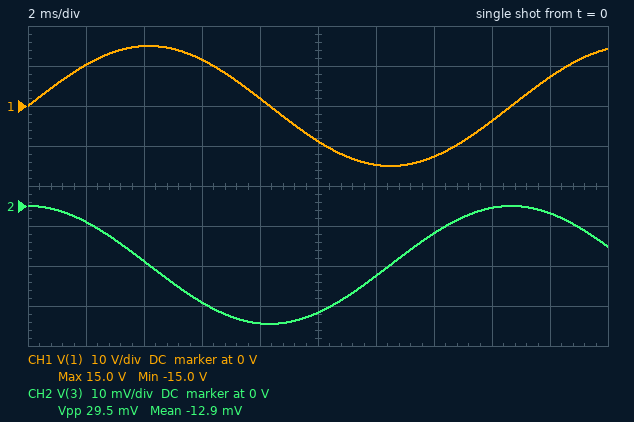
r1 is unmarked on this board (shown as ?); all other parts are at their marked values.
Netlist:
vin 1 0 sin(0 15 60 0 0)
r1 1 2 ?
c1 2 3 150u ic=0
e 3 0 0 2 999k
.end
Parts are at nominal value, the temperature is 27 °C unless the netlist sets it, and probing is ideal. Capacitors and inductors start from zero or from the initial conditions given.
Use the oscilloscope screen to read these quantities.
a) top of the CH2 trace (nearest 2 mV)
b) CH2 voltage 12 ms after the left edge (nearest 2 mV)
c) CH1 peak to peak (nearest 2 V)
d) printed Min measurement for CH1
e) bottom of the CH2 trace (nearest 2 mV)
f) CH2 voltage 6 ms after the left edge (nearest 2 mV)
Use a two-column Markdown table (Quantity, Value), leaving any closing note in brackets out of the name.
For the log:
| Quantity | Value |
|---|---|
| top of the CH2 trace | 0 V |
| CH2 voltage 12 ms after the left edge | -18 mV |
| CH1 peak to peak | 30 V |
| printed Min measurement for CH1 | -15.0 V |
| bottom of the CH2 trace | -30 mV |
| CH2 voltage 6 ms after the left edge | -24 mV |
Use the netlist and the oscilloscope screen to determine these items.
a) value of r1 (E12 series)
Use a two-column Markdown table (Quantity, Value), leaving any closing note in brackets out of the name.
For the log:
| Quantity | Value |
|---|---|
| value of r1 | 18 kΩ |
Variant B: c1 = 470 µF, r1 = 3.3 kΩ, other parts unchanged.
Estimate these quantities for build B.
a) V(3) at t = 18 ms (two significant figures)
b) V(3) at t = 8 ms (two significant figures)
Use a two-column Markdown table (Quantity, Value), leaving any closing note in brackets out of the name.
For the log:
| Quantity | Value |
|---|---|
| V(3) at t = 18 ms | -3.2 mV |
| V(3) at t = 8 ms | -51 mV |
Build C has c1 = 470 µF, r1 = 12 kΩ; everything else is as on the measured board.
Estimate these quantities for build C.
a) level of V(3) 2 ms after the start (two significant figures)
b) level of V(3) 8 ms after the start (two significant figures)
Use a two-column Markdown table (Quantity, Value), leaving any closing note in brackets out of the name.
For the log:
| Quantity | Value |
|---|---|
| level of V(3) 2 ms after the start | -1.9 mV |
| level of V(3) 8 ms after the start | -14 mV |
